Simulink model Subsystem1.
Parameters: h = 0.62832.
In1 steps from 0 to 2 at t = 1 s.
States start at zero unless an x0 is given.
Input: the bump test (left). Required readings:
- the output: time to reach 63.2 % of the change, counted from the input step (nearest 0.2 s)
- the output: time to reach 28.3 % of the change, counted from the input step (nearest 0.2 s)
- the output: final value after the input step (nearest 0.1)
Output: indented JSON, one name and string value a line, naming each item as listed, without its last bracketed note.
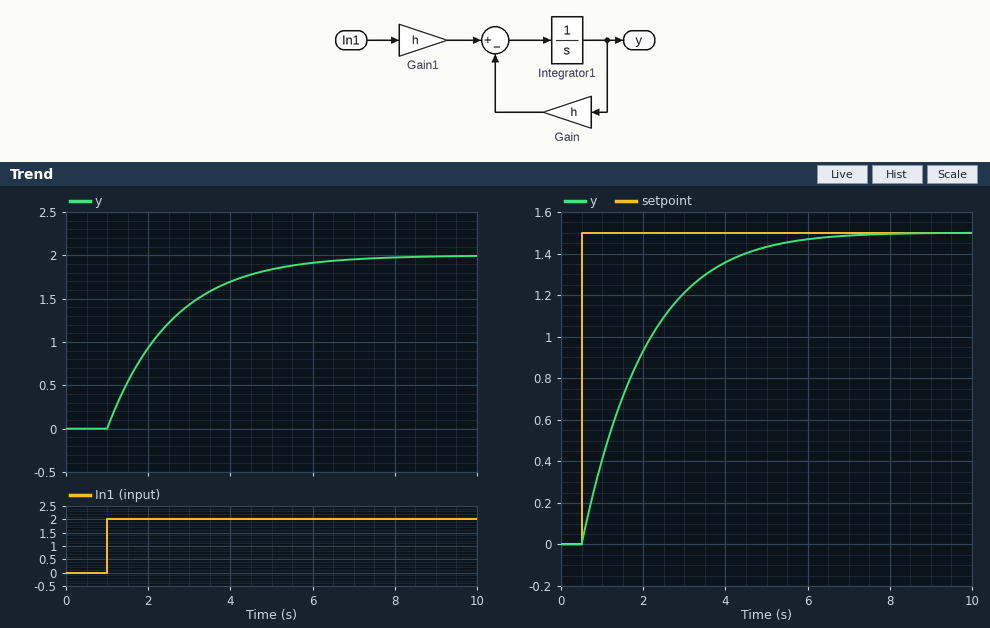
{
  "the output: time to reach 63.2 % of the change, counted from the input step": "1.6 s",
  "the output: time to reach 28.3 % of the change, counted from the input step": "0.6 s",
  "the output: final value after the input step": "2.0"
}
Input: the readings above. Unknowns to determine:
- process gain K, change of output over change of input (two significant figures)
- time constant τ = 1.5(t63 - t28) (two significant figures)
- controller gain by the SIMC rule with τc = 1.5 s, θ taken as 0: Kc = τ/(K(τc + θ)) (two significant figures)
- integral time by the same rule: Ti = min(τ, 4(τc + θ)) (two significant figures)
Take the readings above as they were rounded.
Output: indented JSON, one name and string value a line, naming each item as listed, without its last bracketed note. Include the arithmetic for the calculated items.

{
  "process gain K, change of output over change of input": "(2 - 0) / 2 = 1.0",
  "time constant τ = 1.5(t63 - t28)": "1.5 × (1.6 - 0.6) = 1.5 s",
  "controller gain by the SIMC rule with τc = 1.5 s, θ taken as 0: Kc = τ/(K(τc + θ))": "1.5 / (1 × (1.5 + 0)) = 1.0",
  "integral time by the same rule: Ti = min(τ, 4(τc + θ))": "min(1.5, 4 × (1.5 + 0)) = 1.5 s"
}
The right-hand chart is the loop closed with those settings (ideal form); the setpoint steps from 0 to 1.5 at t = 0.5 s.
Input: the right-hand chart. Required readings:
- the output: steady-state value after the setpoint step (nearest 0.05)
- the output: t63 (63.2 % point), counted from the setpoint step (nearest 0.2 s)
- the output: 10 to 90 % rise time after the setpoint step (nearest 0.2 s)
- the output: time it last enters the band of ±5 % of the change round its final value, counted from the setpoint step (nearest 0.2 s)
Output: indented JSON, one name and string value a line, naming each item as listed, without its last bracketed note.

{
  "the output: steady-state value after the setpoint step": "1.50",
  "the output: t63 (63.2 % point), counted from the setpoint step": "1.6 s",
  "the output: 10 to 90 % rise time after the setpoint step": "3.2 s",
  "the output: time it last enters the band of ±5 % of the change round its final value, counted from the setpoint step": "4.4 s"
}
